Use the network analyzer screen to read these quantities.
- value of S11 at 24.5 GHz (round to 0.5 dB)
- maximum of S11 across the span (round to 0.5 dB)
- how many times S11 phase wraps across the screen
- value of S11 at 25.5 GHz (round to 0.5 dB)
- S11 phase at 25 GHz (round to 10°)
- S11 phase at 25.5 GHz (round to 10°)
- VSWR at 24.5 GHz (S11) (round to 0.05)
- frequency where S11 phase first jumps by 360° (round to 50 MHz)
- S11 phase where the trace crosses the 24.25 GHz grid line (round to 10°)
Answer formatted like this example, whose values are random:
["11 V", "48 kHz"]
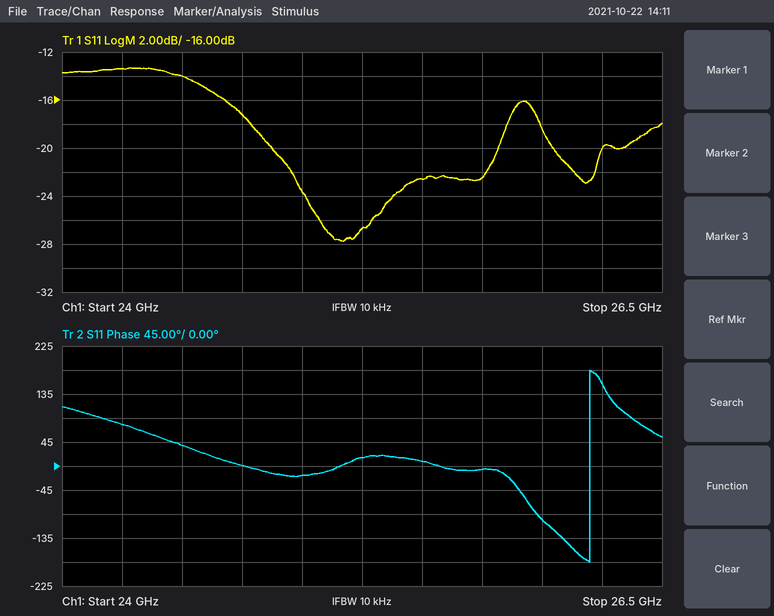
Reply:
["-14.0 dB", "-13.5 dB", "1", "-22.5 dB", "-20°", "10°", "1.50", "26.20 GHz", "80°"]
